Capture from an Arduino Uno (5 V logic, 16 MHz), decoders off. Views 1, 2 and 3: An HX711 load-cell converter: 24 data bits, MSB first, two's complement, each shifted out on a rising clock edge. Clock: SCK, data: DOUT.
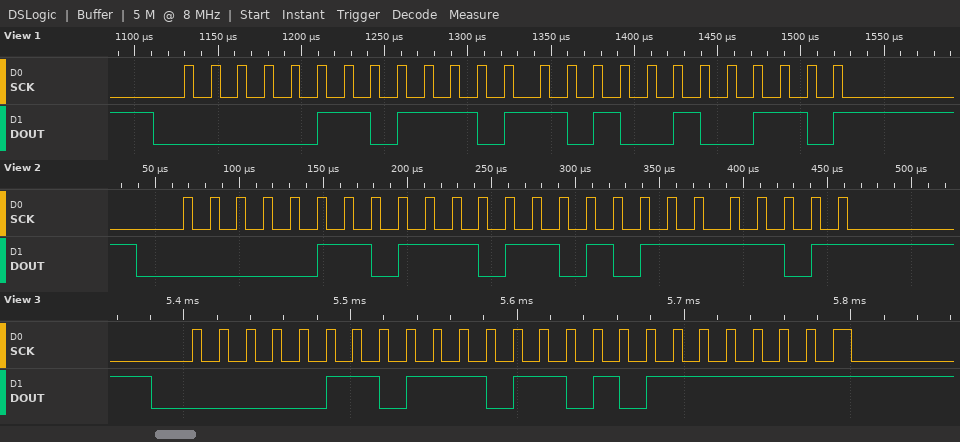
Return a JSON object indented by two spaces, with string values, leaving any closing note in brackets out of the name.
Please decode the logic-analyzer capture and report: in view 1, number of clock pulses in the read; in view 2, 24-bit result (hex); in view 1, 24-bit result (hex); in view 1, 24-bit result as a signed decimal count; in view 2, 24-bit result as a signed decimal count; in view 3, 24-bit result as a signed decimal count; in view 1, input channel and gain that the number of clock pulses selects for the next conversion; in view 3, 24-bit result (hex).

{
  "in view 1, number of clock pulses in the read": "25",
  "in view 2, 24-bit result": "0x06ED7D",
  "in view 1, 24-bit result": "0x06ED26",
  "in view 1, 24-bit result as a signed decimal count": "453926",
  "in view 2, 24-bit result as a signed decimal count": "454013",
  "in view 3, 24-bit result as a signed decimal count": "454015",
  "in view 1, input channel and gain that the number of clock pulses selects for the next conversion": "channel A, gain 128",
  "in view 3, 24-bit result": "0x06ED7F"
}
